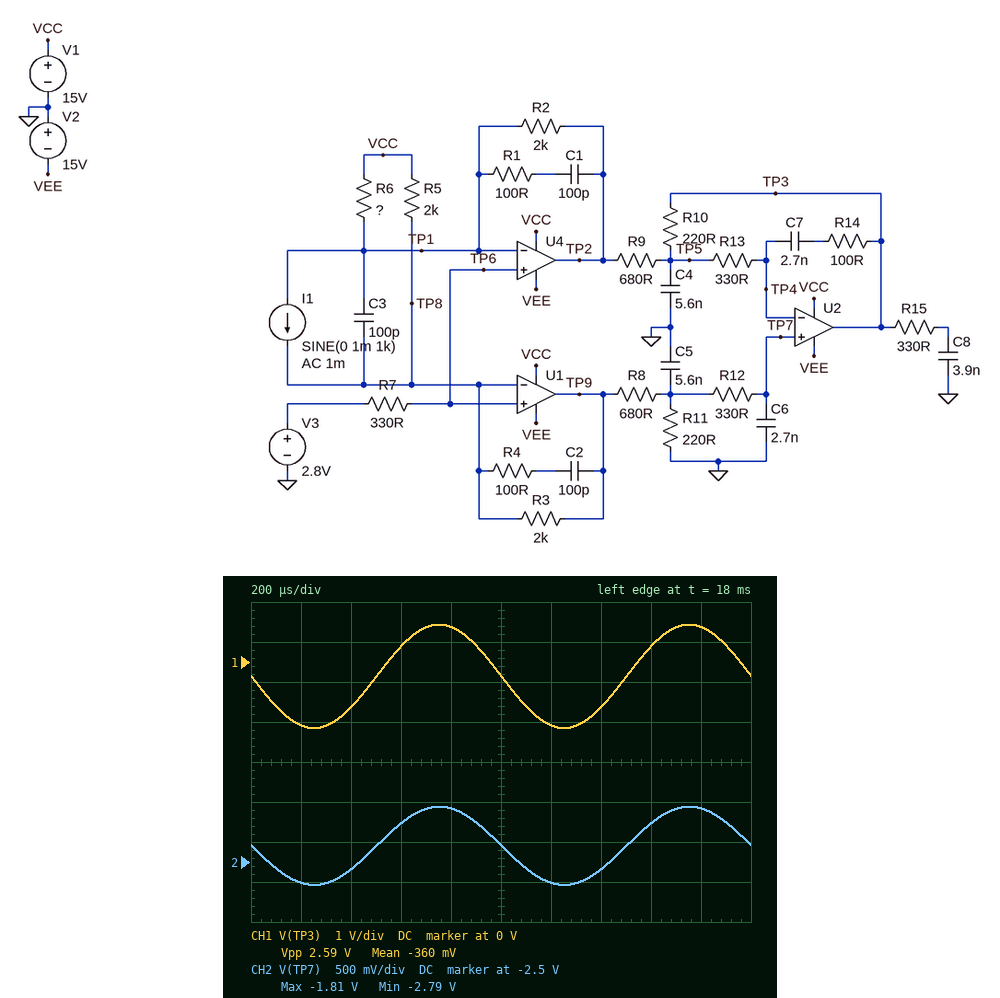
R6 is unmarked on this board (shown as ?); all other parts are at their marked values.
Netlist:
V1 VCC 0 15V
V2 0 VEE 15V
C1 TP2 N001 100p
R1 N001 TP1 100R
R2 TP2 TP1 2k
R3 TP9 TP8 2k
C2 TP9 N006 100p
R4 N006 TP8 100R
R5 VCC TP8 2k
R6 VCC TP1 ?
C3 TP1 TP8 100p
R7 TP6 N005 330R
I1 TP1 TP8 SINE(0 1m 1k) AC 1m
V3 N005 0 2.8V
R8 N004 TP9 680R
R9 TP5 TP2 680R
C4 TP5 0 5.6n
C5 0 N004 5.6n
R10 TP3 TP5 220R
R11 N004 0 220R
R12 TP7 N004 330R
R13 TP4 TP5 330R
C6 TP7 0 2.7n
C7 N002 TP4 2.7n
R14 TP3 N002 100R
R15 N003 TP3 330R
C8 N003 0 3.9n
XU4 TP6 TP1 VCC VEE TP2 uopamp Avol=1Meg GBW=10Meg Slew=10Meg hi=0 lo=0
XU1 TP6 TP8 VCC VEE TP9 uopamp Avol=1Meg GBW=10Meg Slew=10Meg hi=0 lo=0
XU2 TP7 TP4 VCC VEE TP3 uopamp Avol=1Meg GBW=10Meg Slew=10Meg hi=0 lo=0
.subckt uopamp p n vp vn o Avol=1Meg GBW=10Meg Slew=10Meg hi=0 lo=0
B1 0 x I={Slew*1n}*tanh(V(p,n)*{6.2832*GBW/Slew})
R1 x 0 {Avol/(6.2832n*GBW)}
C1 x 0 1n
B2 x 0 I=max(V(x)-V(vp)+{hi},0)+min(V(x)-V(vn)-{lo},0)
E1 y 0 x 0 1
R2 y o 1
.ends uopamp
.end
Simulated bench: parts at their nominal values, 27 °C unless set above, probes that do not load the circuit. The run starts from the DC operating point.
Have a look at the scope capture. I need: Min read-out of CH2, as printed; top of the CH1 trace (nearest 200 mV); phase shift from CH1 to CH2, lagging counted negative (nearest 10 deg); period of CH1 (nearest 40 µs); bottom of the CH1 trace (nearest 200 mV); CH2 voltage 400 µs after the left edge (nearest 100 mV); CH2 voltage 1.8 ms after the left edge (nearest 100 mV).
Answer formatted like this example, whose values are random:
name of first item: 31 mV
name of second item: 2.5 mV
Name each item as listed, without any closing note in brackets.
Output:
Min read-out of CH2, as printed: -2.79 V
top of the CH1 trace: 1.0 V
phase shift from CH1 to CH2, lagging counted negative: 0 deg
period of CH1: 1.00 ms
bottom of the CH1 trace: -1.6 V
CH2 voltage 400 µs after the left edge: -2.6 V
CH2 voltage 1.8 ms after the left edge: -1.8 V
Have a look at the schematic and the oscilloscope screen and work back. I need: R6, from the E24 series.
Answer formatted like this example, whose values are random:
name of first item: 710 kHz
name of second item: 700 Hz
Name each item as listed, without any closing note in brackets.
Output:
R6, from the E24 series: 2.2 kΩ
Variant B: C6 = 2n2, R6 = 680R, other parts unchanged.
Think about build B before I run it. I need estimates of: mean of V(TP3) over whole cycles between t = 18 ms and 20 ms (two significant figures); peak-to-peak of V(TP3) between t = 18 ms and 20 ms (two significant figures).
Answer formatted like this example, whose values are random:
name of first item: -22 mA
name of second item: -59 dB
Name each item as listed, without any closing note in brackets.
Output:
mean of V(TP3) over whole cycles between t = 18 ms and 20 ms: 1.8 V
peak-to-peak of V(TP3) between t = 18 ms and 20 ms: 1.3 V
